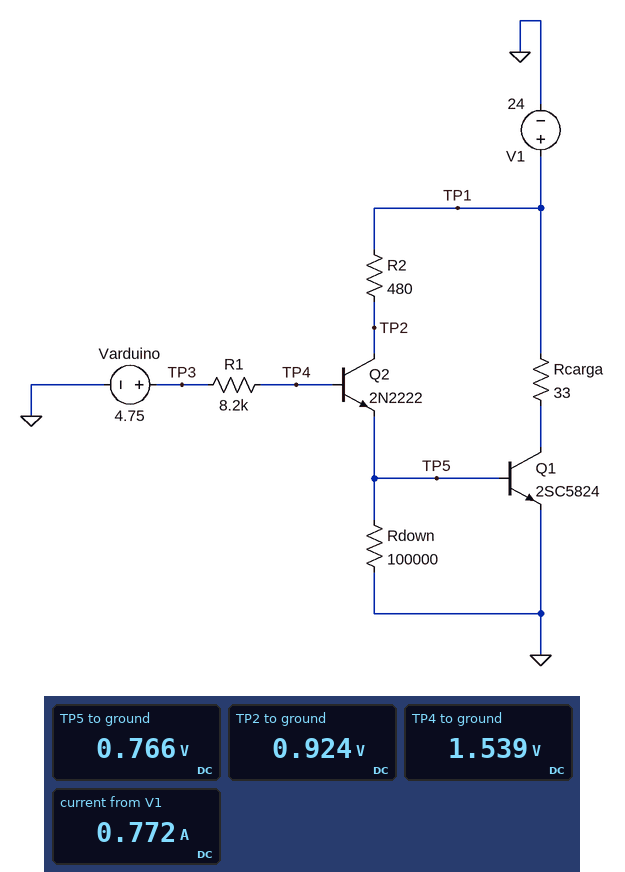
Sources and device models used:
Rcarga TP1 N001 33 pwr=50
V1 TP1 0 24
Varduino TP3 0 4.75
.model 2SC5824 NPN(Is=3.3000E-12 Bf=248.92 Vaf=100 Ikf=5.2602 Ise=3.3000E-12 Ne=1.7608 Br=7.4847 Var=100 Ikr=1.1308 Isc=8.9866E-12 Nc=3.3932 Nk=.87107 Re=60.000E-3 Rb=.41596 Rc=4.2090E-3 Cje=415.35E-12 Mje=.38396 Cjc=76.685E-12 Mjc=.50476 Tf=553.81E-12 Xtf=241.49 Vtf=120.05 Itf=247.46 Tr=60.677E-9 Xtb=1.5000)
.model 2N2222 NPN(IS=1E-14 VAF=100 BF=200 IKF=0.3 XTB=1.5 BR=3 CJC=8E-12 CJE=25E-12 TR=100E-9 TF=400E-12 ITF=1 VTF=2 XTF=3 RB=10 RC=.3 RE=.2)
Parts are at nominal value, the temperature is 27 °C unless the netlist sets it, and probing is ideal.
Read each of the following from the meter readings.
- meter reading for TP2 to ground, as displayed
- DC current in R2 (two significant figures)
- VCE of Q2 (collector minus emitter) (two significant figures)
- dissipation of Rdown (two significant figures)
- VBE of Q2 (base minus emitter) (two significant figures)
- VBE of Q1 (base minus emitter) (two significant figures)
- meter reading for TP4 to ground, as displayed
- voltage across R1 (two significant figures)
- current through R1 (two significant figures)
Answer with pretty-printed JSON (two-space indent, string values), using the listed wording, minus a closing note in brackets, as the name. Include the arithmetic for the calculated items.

{
  "meter reading for TP2 to ground, as displayed": "0.924 V",
  "DC current in R2": "(24 V - 924 mV) / 480 Ω = 48 mA",
  "VCE of Q2 (collector minus emitter)": "924 mV - 766 mV = 160 mV",
  "dissipation of Rdown": "(766 mV)^2 / 100 kΩ = 5.9 µW",
  "VBE of Q2 (base minus emitter)": "1.539 V - 766 mV = 770 mV",
  "VBE of Q1 (base minus emitter)": "766 mV = 770 mV",
  "meter reading for TP4 to ground, as displayed": "1.539 V",
  "voltage across R1": "4.75 V - 1.539 V = 3.2 V",
  "current through R1": "(4.75 V - 1.539 V) / 8.2 kΩ = 390 µA"
}
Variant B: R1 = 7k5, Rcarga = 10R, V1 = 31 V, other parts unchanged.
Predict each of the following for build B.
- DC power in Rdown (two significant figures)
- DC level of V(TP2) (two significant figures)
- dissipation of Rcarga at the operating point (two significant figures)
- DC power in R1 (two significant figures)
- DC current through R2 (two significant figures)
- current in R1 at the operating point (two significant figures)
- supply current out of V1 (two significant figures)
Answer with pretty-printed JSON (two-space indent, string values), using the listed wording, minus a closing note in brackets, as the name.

{
  "DC power in Rdown": "9.3 µW",
  "DC level of V(TP2)": "1.2 V",
  "dissipation of Rcarga at the operating point": "91 W",
  "DC power in R1": "1.2 mW",
  "DC current through R2": "62 mA",
  "current in R1 at the operating point": "400 µA",
  "supply current out of V1": "3.1 A"
}
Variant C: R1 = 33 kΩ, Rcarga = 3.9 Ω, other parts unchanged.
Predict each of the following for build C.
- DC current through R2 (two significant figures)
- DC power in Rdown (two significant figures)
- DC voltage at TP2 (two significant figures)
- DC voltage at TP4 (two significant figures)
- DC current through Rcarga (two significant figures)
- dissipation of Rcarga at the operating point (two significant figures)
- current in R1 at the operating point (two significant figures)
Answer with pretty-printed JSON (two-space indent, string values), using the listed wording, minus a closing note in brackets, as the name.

{
  "DC current through R2": "20 mA",
  "DC power in Rdown": "7.6 µW",
  "DC voltage at TP2": "14 V",
  "DC voltage at TP4": "1.6 V",
  "DC current through Rcarga": "2.3 A",
  "dissipation of Rcarga at the operating point": "21 W",
  "current in R1 at the operating point": "95 µA"
}
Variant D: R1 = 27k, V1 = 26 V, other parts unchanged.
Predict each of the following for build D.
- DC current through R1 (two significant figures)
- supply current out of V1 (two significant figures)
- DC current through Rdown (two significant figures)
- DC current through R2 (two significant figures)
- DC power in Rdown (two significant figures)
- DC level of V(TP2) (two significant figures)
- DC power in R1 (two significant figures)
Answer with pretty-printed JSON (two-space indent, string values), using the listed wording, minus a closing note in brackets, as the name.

{
  "DC current through R1": "120 µA",
  "supply current out of V1": "810 mA",
  "DC current through Rdown": "7.5 µA",
  "DC current through R2": "25 mA",
  "DC power in Rdown": "5.7 µW",
  "DC level of V(TP2)": "14 V",
  "DC power in R1": "390 µW"
}
